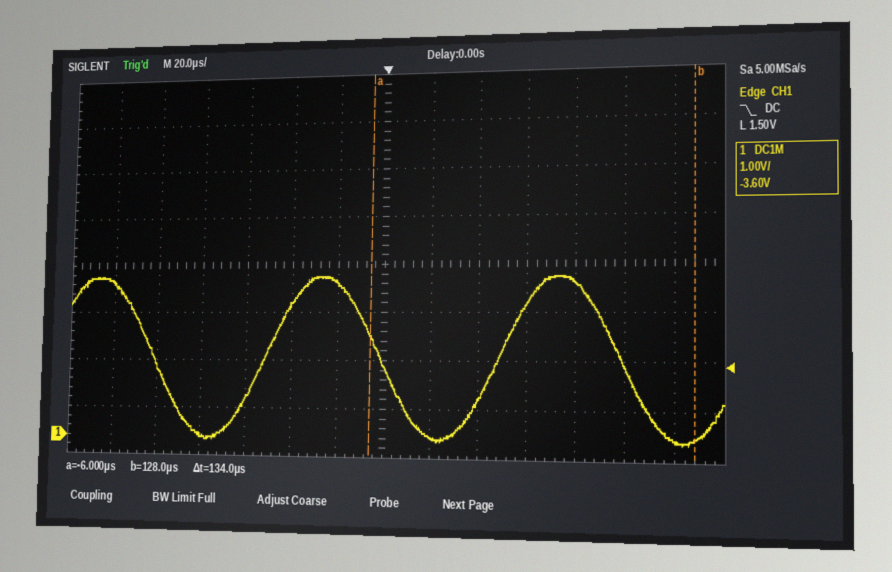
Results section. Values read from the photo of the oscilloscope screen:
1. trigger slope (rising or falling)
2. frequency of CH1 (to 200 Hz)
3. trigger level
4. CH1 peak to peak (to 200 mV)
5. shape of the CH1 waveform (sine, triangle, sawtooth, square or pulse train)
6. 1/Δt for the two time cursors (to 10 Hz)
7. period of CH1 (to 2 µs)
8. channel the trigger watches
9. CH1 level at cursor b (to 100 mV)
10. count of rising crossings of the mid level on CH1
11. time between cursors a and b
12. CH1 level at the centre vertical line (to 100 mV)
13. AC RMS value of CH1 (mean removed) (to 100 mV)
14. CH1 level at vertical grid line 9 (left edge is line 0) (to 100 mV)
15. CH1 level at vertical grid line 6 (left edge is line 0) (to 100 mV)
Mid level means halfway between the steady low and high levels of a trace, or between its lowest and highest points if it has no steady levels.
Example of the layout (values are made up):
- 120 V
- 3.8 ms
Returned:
- falling
- 10.0 kHz
- 1.50 V
- 3.4 V
- sine
- 7.46 kHz
- 100 µs
- CH1
- 100 mV
- 2
- 134 µs
- 1.5 V
- 1.2 V
- 800 mV
- 3.2 V
